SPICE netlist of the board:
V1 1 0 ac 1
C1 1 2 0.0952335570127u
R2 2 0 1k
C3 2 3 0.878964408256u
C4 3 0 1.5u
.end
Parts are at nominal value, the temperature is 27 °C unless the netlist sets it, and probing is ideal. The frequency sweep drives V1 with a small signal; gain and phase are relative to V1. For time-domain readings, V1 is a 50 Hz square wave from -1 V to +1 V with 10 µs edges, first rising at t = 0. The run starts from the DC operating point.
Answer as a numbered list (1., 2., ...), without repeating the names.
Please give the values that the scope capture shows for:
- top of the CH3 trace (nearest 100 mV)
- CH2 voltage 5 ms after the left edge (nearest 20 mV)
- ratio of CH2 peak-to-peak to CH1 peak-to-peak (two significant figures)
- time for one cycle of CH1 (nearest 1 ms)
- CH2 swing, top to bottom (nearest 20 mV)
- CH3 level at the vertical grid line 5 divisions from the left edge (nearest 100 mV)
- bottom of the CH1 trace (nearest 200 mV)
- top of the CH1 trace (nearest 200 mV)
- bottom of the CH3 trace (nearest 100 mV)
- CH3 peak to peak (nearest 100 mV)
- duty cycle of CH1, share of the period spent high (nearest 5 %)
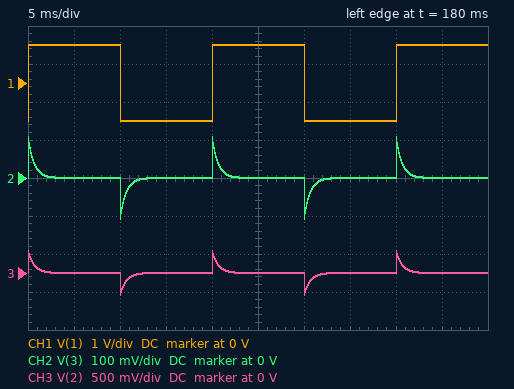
1. 300 mV
2. 0 V
3. 0.11
4. 20 ms
5. 220 mV
6. 0 V
7. -1.0 V
8. 1.0 V
9. -300 mV
10. 600 mV
11. 50 %
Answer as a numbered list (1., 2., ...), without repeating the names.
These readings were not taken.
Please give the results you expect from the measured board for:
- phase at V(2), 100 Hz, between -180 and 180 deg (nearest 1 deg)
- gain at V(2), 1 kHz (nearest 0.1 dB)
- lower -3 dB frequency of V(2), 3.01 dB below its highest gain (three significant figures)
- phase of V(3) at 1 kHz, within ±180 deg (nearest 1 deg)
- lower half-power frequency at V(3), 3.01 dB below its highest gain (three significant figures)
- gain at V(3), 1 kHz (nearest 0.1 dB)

1. 68 deg
2. -16.9 dB
3. 245 Hz
4. 14 deg
5. 245 Hz
6. -25.6 dB
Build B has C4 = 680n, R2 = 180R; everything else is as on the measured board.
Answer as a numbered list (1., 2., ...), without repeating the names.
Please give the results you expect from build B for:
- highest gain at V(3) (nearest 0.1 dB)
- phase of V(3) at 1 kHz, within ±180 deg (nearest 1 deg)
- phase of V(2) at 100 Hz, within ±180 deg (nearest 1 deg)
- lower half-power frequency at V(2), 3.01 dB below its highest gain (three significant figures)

1. -19.0 dB
2. 62 deg
3. 87 deg
4. 1.85 kHz
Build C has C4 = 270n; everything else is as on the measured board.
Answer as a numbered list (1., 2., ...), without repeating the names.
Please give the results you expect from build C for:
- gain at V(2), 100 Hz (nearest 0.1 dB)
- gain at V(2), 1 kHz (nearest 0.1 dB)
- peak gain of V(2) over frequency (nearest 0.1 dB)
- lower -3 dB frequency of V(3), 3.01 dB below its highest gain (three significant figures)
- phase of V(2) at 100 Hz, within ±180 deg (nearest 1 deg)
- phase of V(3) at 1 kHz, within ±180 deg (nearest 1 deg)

1. -24.6 dB
2. -11.1 dB
3. -10.0 dB
4. 527 Hz
5. 79 deg
6. 28 deg
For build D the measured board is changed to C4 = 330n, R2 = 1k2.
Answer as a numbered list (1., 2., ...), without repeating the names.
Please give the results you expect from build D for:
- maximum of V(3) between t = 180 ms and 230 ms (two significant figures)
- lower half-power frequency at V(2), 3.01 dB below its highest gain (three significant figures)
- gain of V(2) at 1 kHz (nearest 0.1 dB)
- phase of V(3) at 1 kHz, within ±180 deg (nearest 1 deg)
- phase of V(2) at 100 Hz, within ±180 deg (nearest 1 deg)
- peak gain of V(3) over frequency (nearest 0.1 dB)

1. 410 mV
2. 396 Hz
3. -11.6 dB
4. 22 deg
5. 76 deg
6. -13.7 dB
